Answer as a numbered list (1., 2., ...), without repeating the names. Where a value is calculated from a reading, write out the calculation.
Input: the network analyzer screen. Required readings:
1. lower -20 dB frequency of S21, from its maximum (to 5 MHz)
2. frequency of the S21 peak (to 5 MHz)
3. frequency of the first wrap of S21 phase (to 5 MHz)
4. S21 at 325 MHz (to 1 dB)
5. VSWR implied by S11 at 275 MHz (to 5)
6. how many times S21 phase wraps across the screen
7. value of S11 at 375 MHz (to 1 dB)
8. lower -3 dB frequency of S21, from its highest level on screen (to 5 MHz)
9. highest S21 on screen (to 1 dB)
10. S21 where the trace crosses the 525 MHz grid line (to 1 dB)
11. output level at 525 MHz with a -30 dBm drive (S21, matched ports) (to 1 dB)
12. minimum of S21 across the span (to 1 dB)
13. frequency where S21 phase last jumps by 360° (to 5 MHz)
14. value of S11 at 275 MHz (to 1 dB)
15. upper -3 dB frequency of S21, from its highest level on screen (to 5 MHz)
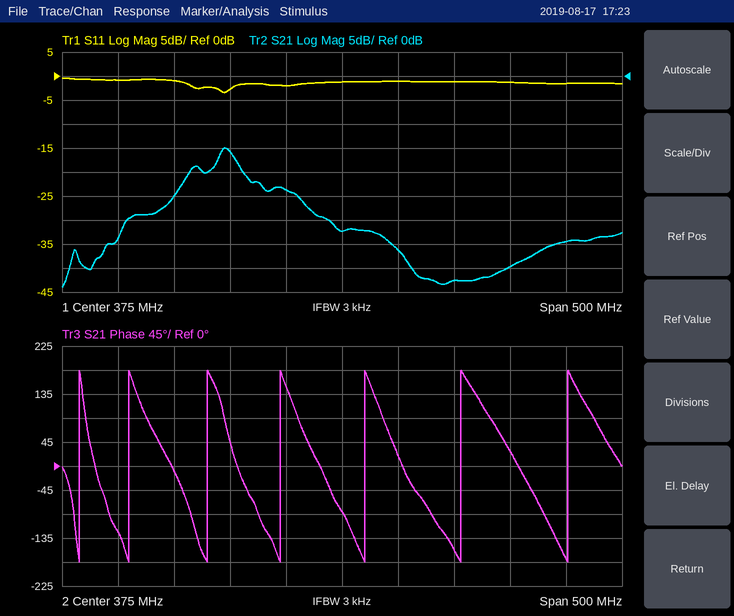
1. 170 MHz
2. 270 MHz
3. 140 MHz
4. -24 dB
5. |Γ| = 10^(-3/20) = 0.7079; VSWR = (1 + 0.7079)/(1 − 0.7079) ≈ 5.85, so 5 to the nearest 5
6. 7
7. -1 dB
8. 265 MHz
9. -15 dB
10. -40 dB
11. -30 dBm + (-40 dB) = -70 dBm
12. -44 dB
13. 575 MHz
14. -3 dB
15. 280 MHz
